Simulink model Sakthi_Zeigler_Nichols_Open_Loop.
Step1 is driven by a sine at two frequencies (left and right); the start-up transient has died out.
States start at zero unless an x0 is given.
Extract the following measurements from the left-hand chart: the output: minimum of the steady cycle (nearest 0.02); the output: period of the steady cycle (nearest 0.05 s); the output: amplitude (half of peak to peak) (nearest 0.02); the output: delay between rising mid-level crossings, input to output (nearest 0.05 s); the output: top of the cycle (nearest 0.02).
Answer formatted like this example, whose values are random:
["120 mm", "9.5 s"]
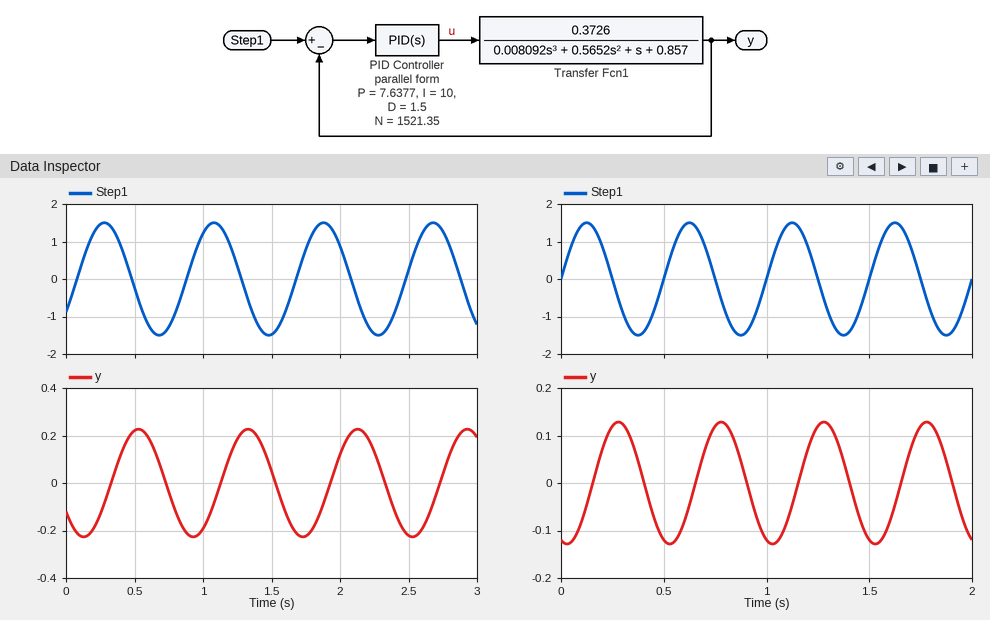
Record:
["-0.22", "0.80 s", "0.22", "0.25 s", "0.22"]
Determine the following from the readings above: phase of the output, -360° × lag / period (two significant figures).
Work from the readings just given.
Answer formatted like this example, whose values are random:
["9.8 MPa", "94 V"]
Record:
["-110°"]
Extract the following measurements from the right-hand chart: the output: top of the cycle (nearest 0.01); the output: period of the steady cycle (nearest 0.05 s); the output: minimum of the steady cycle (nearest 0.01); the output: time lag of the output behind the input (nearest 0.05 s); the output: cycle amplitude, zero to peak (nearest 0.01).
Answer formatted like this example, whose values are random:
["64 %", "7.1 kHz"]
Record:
["0.13", "0.50 s", "-0.13", "0.15 s", "0.13"]
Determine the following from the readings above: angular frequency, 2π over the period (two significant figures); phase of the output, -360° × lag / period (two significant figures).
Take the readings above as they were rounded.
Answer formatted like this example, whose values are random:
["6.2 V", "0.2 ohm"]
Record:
["13 rad/s", "-110°"]
